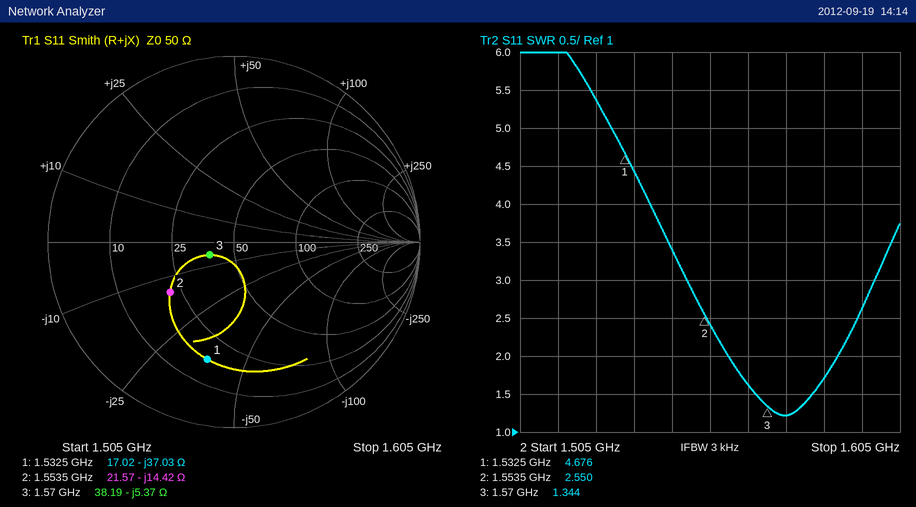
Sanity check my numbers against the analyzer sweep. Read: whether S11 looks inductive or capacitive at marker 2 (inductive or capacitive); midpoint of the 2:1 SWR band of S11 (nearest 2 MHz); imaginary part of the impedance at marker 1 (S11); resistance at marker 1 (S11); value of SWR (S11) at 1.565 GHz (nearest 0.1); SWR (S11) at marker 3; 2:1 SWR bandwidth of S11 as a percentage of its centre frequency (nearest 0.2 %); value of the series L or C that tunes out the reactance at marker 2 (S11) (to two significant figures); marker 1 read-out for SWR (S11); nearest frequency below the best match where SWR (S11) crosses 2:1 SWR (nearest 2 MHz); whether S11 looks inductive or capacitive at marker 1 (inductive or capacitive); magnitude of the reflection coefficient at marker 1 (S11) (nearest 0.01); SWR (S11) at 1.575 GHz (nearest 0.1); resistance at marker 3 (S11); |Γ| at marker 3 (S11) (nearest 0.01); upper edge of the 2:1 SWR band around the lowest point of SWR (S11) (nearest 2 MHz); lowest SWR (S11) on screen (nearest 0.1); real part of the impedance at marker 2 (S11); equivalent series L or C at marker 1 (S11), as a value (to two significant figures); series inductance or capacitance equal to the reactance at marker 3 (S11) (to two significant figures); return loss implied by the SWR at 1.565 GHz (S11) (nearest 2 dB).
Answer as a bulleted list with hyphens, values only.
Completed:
- capacitive
- 1.574 GHz
- -37.03 Ω
- 17.02 Ω
- 1.6
- 1.344
- 1.8 %
- 1.5 nH
- 4.676
- 1.560 GHz
- capacitive
- 0.65
- 1.2
- 38.19 Ω
- 0.15
- 1.588 GHz
- 1.2
- 21.57 Ω
- 2.8 pF
- 19 pF
- 12 dB
